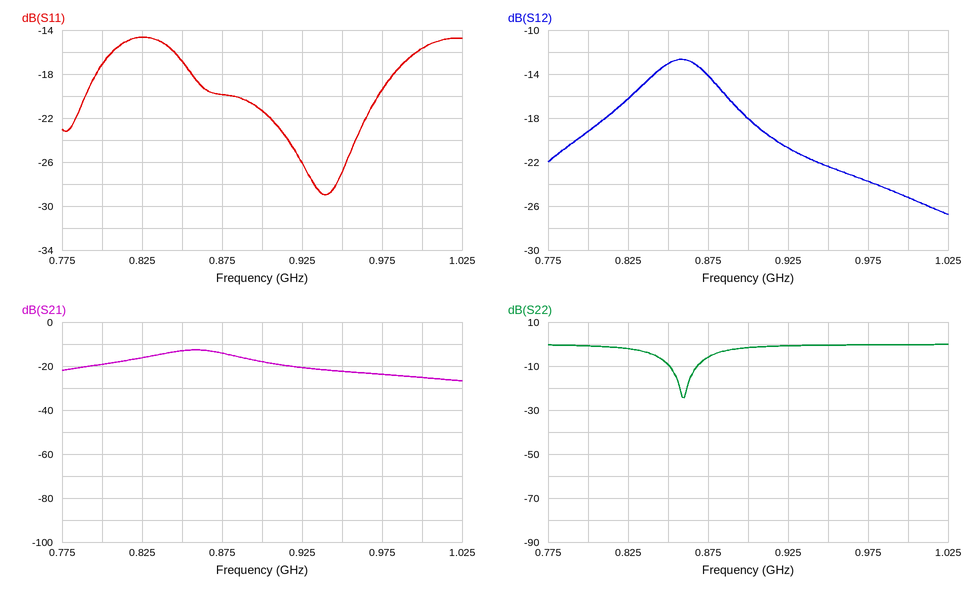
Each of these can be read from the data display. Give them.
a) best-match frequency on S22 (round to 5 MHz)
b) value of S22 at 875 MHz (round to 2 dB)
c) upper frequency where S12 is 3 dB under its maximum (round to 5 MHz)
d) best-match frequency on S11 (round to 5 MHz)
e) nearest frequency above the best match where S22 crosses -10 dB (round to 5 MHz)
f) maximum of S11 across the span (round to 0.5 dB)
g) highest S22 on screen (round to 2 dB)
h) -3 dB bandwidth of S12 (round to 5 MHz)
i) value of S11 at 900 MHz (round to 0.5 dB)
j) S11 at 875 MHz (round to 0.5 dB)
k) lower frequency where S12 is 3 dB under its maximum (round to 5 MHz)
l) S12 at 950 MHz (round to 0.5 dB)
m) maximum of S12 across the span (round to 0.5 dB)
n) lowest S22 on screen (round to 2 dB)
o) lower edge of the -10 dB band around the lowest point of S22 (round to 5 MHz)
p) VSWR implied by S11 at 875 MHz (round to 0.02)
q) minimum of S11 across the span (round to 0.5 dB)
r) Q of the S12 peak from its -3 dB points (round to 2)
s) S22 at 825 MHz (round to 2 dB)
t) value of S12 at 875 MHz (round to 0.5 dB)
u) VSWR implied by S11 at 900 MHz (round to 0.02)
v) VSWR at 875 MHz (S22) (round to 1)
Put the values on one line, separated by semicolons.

860 MHz; -6 dB; 885 MHz; 940 MHz; 870 MHz; -14.5 dB; 0 dB; 55 MHz; -21.5 dB; -20.0 dB; 830 MHz; -22.5 dB; -12.5 dB; -24 dB; 850 MHz; 1.22; -29.0 dB; 16; -2 dB; -14.0 dB; 1.18; 3
